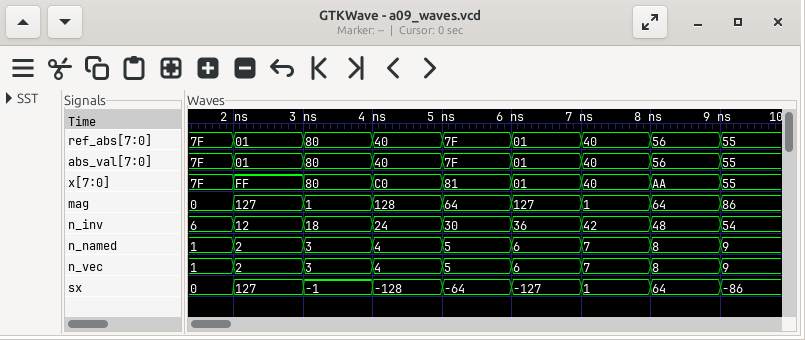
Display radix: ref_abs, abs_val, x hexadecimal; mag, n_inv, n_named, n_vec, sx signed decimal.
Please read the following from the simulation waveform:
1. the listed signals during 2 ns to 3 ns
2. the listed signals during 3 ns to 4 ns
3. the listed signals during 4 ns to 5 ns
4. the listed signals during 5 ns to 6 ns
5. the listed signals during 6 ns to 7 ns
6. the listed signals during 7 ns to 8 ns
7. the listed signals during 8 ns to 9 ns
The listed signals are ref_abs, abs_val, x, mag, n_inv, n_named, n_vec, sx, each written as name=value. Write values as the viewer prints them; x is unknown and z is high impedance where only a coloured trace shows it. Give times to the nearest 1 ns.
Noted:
ref_abs=01, abs_val=01, x=FF, mag=127, n_inv=12, n_named=2, n_vec=2, sx=127
ref_abs=80, abs_val=80, x=80, mag=1, n_inv=18, n_named=3, n_vec=3, sx=-1
ref_abs=40, abs_val=40, x=C0, mag=128, n_inv=24, n_named=4, n_vec=4, sx=-128
ref_abs=7F, abs_val=7F, x=81, mag=64, n_inv=30, n_named=5, n_vec=5, sx=-64
ref_abs=01, abs_val=01, x=01, mag=127, n_inv=36, n_named=6, n_vec=6, sx=-127
ref_abs=40, abs_val=40, x=40, mag=1, n_inv=42, n_named=7, n_vec=7, sx=1
ref_abs=56, abs_val=56, x=AA, mag=64, n_inv=48, n_named=8, n_vec=8, sx=64
